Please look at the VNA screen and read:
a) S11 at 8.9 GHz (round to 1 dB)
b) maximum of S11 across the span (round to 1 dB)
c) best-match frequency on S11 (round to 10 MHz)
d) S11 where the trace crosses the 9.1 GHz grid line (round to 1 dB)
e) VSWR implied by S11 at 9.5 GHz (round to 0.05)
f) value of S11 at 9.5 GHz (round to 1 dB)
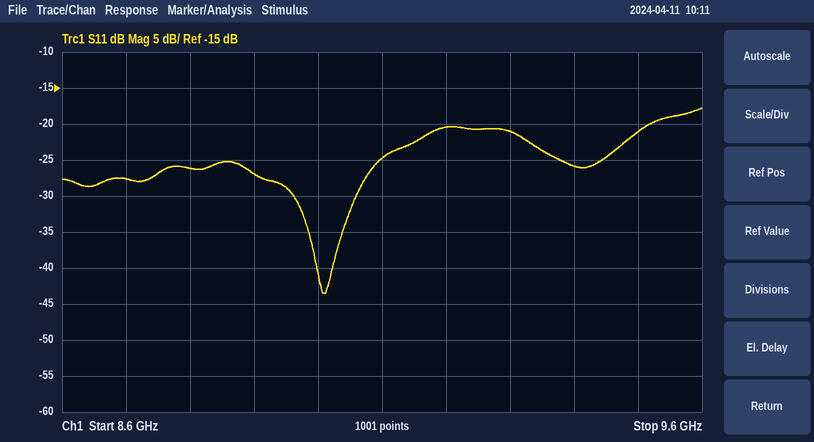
-27 dB
-18 dB
9.01 GHz
-25 dB
1.20
-21 dB
